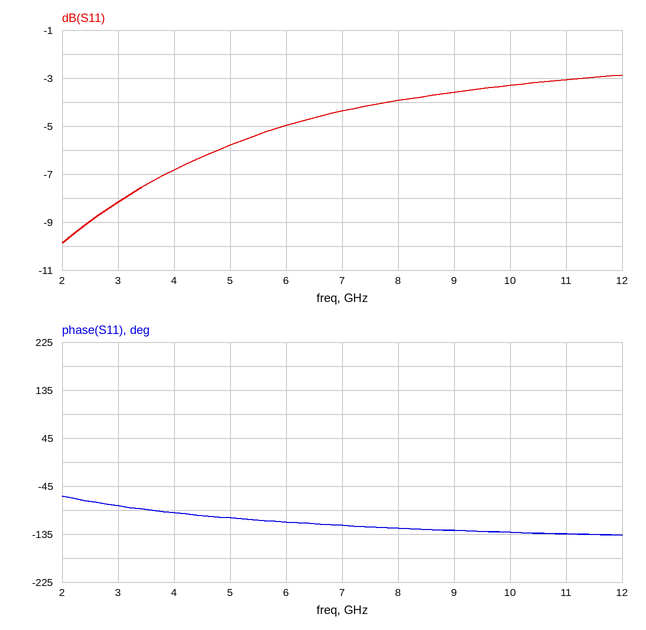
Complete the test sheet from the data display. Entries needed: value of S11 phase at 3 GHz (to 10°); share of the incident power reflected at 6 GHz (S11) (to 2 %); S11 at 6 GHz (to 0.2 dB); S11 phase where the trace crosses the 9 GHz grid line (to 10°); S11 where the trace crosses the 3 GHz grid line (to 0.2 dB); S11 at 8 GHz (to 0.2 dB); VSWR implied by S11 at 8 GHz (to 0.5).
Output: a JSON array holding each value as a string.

["-80°", "32 %", "-5.0 dB", "-130°", "-8.2 dB", "-4.0 dB", "4.5"]
